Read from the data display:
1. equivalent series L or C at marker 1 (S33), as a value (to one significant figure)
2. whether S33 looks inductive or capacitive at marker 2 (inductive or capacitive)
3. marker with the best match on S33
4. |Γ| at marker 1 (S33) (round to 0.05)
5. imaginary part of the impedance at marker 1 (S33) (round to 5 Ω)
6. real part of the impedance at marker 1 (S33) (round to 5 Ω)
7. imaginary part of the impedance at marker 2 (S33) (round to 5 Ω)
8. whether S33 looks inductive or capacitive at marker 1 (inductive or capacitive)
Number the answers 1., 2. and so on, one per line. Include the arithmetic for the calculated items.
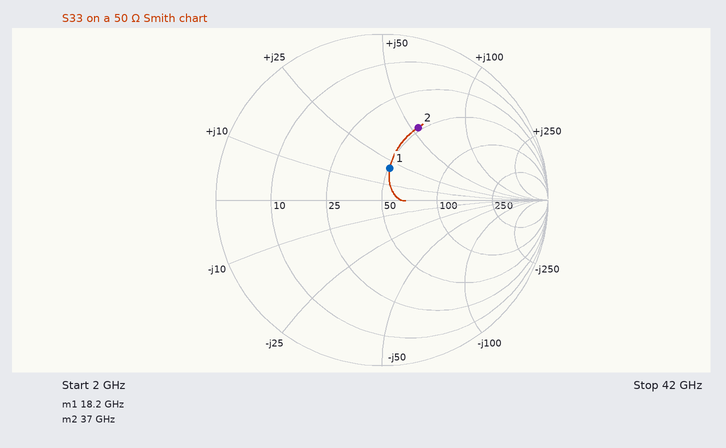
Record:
1. L = 20 Ω/(2π × 18.2 GHz) ≈ 175 pH, so 200 pH to one significant figure
2. inductive
3. marker 1
4. 0.20
5. +20 Ω
6. 50 Ω
7. +55 Ω
8. inductive
